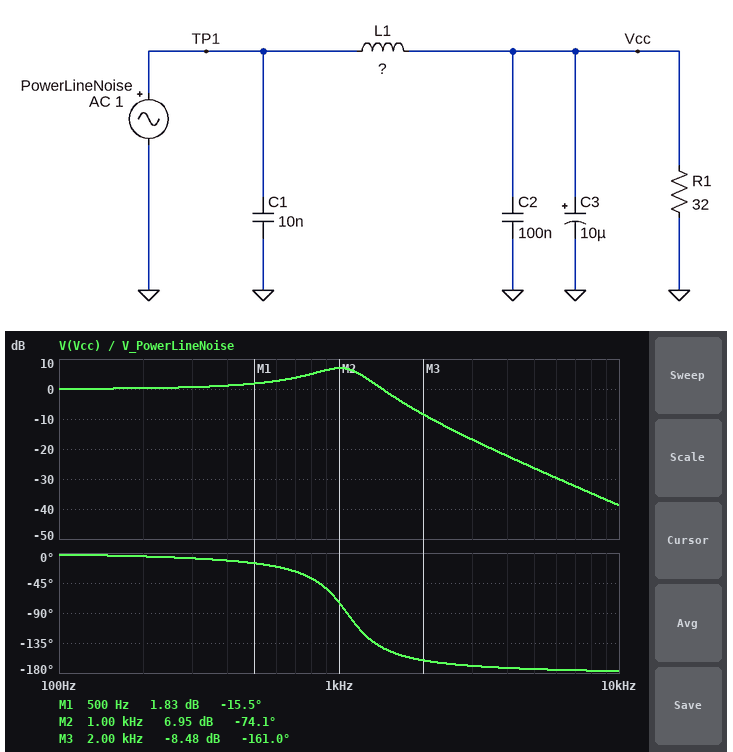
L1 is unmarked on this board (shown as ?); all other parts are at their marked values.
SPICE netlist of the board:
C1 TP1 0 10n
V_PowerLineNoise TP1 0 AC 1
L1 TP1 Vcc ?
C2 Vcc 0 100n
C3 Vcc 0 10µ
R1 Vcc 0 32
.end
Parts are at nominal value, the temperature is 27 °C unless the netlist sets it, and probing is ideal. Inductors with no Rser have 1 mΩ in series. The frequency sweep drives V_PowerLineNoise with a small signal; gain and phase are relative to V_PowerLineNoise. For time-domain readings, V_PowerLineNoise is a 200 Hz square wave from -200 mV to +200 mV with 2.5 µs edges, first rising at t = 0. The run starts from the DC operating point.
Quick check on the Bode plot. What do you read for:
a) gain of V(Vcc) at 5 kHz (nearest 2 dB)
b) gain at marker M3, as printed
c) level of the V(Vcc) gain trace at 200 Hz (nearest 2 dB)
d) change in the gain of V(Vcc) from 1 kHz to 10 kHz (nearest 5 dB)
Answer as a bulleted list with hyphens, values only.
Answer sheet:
- -26 dB
- -8.48 dB
- 0 dB
- -45 dB
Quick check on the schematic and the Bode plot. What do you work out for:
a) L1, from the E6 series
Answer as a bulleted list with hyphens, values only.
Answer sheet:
- 2.2 mH
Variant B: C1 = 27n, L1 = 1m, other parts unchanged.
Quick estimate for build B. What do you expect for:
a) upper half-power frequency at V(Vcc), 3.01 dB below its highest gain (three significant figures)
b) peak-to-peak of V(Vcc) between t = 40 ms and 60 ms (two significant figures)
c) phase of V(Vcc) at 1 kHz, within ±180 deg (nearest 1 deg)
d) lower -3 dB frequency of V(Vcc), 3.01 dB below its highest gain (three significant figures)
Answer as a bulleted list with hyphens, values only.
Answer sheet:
- 1.78 kHz
- 880 mV
- -18 deg
- 1.27 kHz
